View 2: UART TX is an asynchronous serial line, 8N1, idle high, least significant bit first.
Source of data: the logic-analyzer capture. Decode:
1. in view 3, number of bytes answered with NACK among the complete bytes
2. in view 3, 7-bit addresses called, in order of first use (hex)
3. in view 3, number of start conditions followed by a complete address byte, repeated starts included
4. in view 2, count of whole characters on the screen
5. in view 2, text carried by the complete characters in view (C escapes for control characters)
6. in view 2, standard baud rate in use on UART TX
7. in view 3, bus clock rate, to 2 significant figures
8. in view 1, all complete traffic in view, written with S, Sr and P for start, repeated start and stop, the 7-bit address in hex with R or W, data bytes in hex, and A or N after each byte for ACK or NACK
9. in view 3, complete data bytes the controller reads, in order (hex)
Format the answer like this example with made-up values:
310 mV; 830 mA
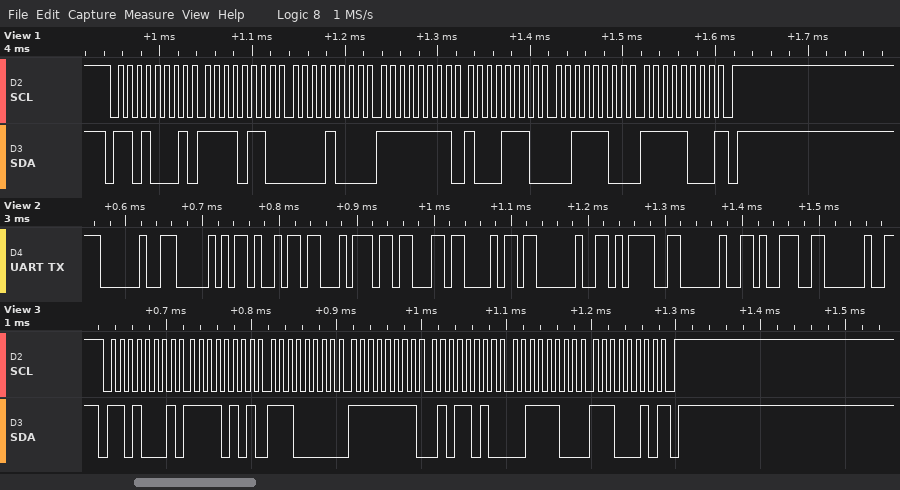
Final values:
1; 0x68; 1; 11; " Pitch = 9 "; 115200 baud; 100 kHz; S 68R A F6 A 08 A FF A 8E A 3C A F8 N P; F5 E0 FF 5A 3C E2
